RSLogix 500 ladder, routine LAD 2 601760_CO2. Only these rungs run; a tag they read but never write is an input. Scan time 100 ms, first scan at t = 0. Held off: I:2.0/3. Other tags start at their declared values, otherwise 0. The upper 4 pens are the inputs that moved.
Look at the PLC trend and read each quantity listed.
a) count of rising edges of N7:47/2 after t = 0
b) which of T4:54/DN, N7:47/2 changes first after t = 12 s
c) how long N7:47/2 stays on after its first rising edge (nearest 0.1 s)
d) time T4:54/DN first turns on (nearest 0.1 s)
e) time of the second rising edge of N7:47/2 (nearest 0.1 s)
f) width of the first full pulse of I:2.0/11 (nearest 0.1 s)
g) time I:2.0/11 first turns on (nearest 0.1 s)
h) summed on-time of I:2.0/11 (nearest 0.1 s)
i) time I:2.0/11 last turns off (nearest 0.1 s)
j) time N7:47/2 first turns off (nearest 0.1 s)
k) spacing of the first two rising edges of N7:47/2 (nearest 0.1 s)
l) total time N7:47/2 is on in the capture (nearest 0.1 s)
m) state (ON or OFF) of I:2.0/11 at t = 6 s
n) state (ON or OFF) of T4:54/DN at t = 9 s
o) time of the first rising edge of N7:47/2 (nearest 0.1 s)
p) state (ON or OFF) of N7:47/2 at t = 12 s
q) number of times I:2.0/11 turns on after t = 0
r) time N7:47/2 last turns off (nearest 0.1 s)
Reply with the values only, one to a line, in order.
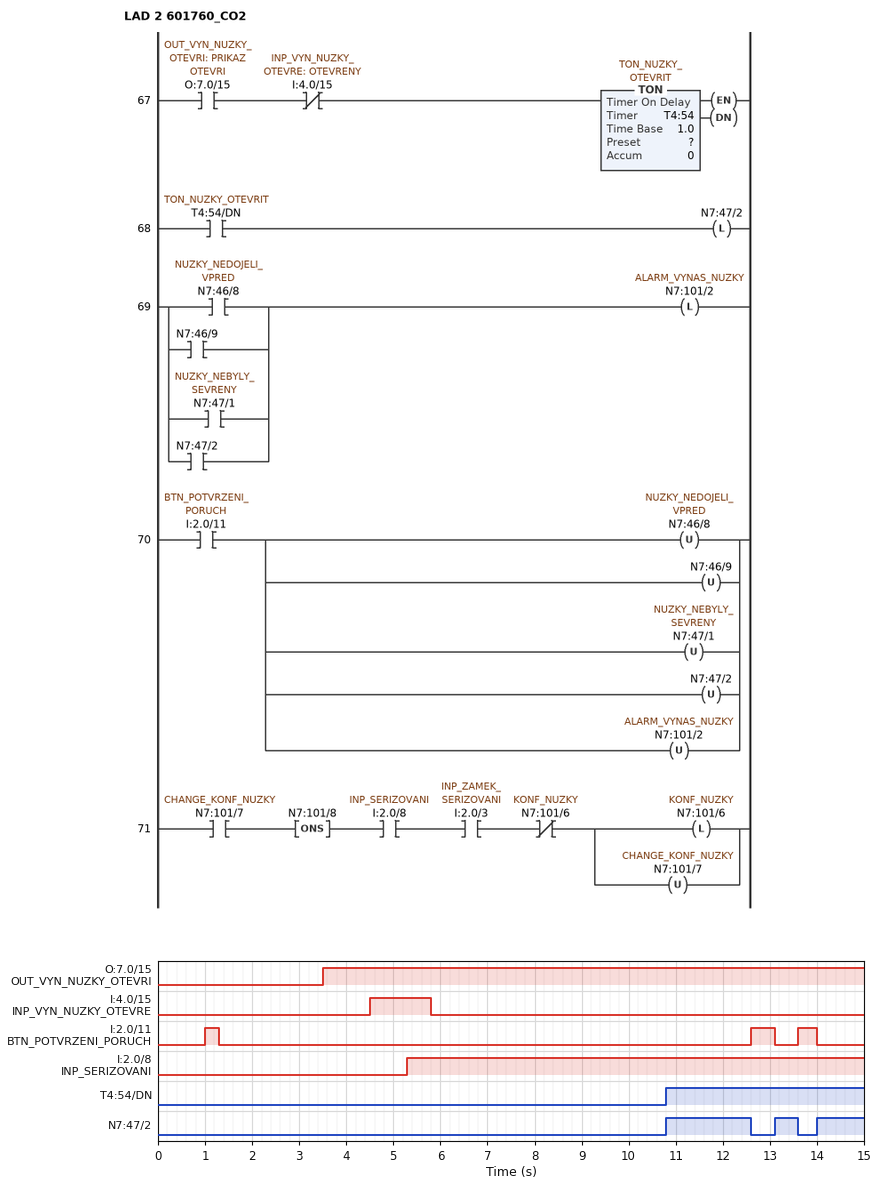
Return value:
3
N7:47/2
1.8 s
10.8 s
13.1 s
0.3 s
1.0 s
1.2 s
14.0 s
12.6 s
2.3 s
3.3 s
OFF
OFF
10.8 s
ON
3
13.6 s
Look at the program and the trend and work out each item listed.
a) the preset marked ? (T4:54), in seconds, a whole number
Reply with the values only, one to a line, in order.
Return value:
5 s
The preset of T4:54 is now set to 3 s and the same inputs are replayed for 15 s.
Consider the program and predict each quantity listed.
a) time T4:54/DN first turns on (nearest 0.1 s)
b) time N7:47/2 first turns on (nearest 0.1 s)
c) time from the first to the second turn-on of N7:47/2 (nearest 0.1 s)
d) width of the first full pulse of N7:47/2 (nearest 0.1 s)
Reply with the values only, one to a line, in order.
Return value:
8.8 s
8.8 s
4.3 s
3.8 s
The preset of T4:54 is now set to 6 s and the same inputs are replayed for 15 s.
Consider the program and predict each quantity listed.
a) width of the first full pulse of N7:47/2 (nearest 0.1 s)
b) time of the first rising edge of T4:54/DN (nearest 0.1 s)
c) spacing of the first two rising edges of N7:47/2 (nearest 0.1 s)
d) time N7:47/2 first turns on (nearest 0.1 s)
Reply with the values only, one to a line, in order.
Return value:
0.8 s
11.8 s
1.3 s
11.8 s
